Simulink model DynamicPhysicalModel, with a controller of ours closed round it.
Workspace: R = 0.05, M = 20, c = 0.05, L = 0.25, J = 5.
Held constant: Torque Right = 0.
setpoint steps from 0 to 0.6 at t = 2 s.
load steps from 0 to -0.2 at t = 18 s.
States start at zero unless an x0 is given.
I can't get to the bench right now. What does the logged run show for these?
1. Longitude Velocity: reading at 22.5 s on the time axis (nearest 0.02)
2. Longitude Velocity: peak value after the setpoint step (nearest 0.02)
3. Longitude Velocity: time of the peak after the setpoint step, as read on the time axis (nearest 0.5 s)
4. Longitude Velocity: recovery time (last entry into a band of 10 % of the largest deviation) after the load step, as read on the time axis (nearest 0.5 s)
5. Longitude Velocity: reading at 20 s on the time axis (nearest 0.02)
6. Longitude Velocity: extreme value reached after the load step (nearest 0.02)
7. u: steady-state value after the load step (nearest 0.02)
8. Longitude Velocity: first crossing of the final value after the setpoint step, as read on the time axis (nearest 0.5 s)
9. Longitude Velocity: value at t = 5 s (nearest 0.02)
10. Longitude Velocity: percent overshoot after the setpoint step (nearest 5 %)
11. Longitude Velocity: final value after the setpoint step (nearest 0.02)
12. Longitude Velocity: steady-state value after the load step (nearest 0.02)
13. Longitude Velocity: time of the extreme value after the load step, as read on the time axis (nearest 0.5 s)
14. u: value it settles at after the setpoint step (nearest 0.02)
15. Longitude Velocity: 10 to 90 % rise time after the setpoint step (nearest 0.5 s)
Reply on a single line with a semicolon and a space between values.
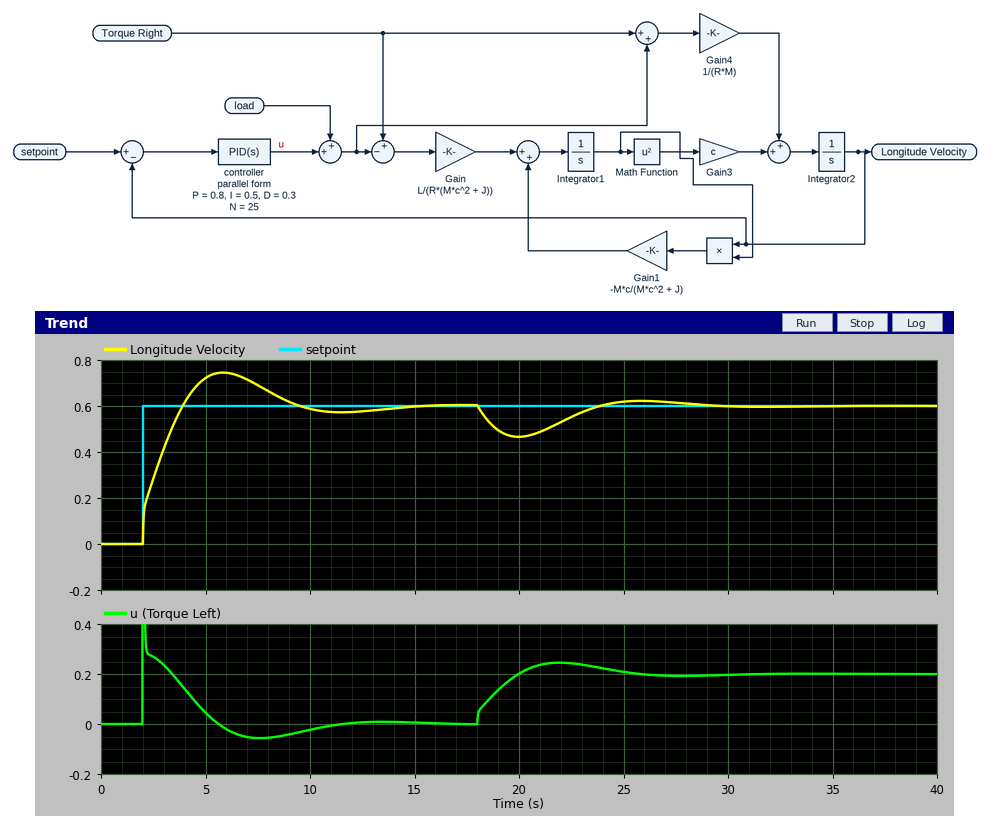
0.56; 0.74; 6.0 s; 27.5 s; 0.46; 0.46; 0.20; 4.0 s; 0.72; 25 %; 0.60; 0.60; 20.0 s; 0.00; 1.5 s
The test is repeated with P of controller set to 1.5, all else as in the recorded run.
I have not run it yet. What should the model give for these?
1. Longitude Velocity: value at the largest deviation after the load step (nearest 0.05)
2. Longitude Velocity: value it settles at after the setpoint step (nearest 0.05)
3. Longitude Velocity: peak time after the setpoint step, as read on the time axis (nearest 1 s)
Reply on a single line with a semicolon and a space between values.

0.50; 0.60; 5 s
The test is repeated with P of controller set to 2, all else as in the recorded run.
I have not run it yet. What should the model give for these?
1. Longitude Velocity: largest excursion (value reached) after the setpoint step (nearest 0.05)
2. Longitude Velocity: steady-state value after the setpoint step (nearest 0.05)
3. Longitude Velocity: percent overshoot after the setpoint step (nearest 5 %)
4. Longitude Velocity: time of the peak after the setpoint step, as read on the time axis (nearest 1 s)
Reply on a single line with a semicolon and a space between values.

0.65; 0.60; 10 %; 5 s
